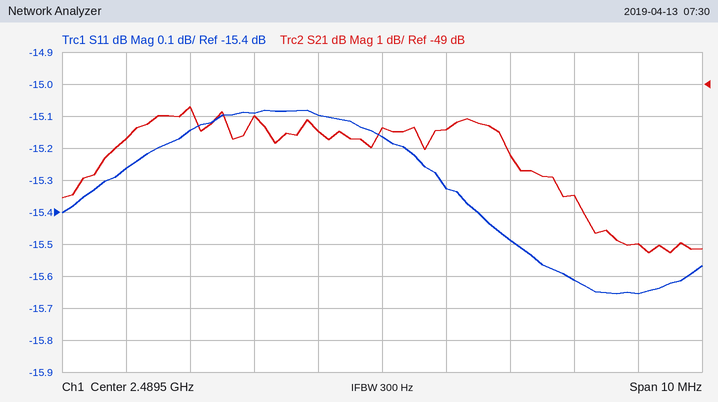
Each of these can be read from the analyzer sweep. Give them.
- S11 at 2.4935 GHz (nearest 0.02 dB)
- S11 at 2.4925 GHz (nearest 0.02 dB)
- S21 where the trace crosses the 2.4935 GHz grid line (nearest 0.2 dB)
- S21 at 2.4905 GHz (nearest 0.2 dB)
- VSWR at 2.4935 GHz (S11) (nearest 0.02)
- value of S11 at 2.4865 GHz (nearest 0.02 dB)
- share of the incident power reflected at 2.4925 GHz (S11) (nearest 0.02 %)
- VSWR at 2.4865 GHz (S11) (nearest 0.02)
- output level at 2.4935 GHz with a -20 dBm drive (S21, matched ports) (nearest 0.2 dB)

-15.66 dB
-15.62 dB
-54.0 dB
-50.4 dB
1.40
-15.14 dB
2.74 %
1.42
-74.0 dBm
